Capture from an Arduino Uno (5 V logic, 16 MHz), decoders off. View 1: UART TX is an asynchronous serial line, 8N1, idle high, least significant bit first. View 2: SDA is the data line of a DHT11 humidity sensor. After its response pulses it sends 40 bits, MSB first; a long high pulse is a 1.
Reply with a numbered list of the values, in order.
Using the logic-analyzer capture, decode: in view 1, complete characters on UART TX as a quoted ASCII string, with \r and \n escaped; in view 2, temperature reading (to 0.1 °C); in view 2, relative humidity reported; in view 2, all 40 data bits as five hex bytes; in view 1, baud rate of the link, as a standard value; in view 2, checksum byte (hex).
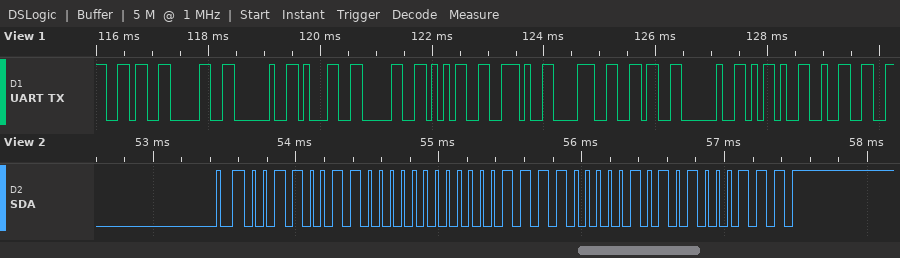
1. "60 105.86 -2"
2. 15.5 °C
3. 51 %
4. 33 00 0F 05 47
5. 9600 baud
6. 0x47
